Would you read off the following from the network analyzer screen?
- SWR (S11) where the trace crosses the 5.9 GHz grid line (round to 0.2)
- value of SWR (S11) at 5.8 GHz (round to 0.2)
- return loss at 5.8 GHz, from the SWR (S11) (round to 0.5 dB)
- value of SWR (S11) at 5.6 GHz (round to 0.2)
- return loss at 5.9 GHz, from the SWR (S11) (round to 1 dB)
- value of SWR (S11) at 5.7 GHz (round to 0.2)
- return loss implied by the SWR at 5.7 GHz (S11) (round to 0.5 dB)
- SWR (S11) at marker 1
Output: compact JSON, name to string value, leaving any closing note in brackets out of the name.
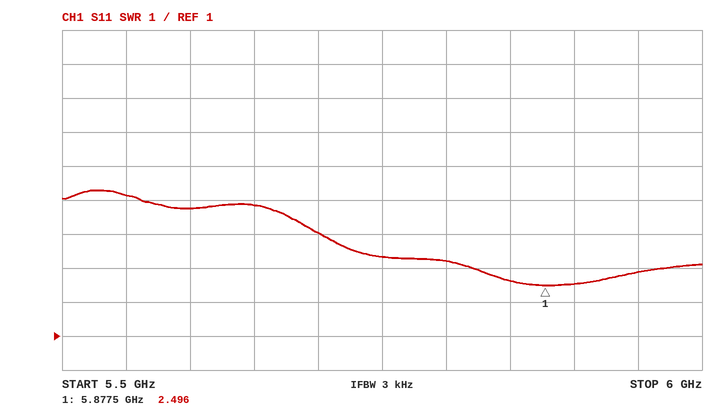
{"SWR (S11) where the trace crosses the 5.9 GHz grid line": "2.6", "value of SWR (S11) at 5.8 GHz": "3.2", "return loss at 5.8 GHz, from the SWR (S11)": "5.5 dB", "value of SWR (S11) at 5.6 GHz": "4.8", "return loss at 5.9 GHz, from the SWR (S11)": "7 dB", "value of SWR (S11) at 5.7 GHz": "4.0", "return loss implied by the SWR at 5.7 GHz (S11)": "4.5 dB", "SWR (S11) at marker 1": "2.496"}
